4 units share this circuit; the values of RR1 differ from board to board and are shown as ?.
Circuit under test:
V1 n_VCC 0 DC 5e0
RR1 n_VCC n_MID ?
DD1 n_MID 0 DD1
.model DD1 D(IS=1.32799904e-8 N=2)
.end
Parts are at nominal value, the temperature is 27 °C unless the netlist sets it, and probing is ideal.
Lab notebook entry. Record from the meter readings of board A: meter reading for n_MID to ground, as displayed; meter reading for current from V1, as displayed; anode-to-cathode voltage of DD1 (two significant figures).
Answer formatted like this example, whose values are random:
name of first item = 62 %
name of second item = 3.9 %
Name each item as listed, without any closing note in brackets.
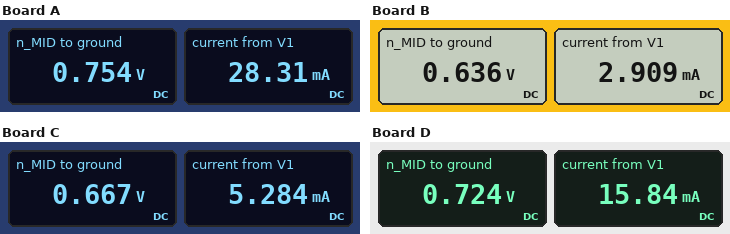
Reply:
meter reading for n_MID to ground, as displayed = 0.754 V
meter reading for current from V1, as displayed = 28.31 mA
anode-to-cathode voltage of DD1 = 750 mV
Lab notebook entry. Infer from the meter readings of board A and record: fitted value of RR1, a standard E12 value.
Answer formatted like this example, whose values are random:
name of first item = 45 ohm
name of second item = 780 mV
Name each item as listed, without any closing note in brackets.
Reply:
fitted value of RR1, a standard E12 value = 150 Ω
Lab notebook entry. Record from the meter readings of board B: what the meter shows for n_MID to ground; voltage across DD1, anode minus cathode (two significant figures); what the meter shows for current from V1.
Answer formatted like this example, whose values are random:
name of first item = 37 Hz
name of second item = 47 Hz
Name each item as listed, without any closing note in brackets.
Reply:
what the meter shows for n_MID to ground = 0.636 V
voltage across DD1, anode minus cathode = 640 mV
what the meter shows for current from V1 = 2.909 mA
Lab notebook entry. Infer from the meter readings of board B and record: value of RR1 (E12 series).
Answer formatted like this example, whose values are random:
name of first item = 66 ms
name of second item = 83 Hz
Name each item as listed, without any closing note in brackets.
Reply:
value of RR1 = 1.5 kΩ
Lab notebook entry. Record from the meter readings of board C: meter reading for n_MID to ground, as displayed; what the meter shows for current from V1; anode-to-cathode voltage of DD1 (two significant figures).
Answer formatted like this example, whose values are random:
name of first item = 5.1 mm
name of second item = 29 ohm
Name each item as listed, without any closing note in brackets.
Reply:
meter reading for n_MID to ground, as displayed = 0.667 V
what the meter shows for current from V1 = 5.284 mA
anode-to-cathode voltage of DD1 = 670 mV
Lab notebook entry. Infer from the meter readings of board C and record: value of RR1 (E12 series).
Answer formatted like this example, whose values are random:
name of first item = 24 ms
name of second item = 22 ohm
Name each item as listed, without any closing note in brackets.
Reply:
value of RR1 = 820 Ω
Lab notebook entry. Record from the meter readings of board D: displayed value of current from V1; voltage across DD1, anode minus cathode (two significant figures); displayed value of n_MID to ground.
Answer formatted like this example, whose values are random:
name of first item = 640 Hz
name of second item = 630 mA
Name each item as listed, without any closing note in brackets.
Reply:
displayed value of current from V1 = 15.84 mA
voltage across DD1, anode minus cathode = 720 mV
displayed value of n_MID to ground = 0.724 V
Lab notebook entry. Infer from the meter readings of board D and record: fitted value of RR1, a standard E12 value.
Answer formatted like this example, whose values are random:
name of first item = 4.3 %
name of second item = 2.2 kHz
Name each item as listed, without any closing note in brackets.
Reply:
fitted value of RR1, a standard E12 value = 270 Ω
